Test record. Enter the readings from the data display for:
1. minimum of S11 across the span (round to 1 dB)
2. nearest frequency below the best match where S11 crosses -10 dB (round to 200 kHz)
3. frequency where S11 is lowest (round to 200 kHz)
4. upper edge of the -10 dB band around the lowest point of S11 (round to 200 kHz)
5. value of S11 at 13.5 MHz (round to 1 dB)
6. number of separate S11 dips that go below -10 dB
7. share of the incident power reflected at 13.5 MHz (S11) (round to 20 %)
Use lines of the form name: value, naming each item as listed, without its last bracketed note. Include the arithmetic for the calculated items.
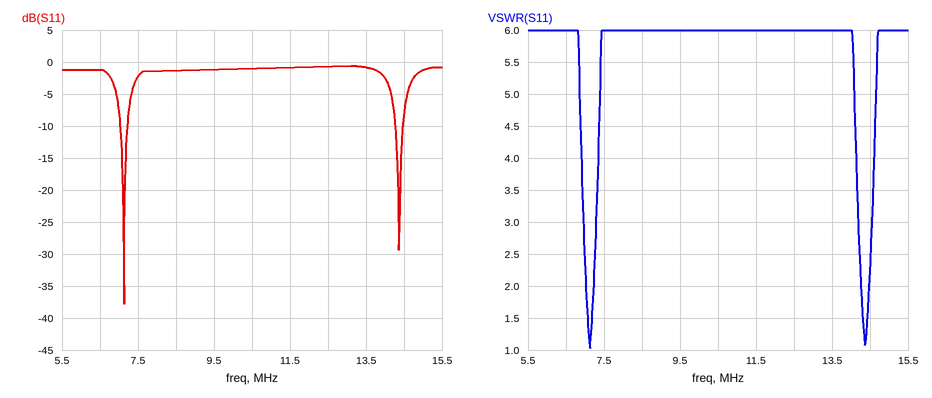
minimum of S11 across the span: -38 dB
nearest frequency below the best match where S11 crosses -10 dB: 7.0 MHz
frequency where S11 is lowest: 7.2 MHz
upper edge of the -10 dB band around the lowest point of S11: 7.2 MHz
value of S11 at 13.5 MHz: -1 dB
number of separate S11 dips that go below -10 dB: 2
share of the incident power reflected at 13.5 MHz (S11): 10^(-1/10) ≈ 79.4 %, so 80 % to the nearest 20 %
